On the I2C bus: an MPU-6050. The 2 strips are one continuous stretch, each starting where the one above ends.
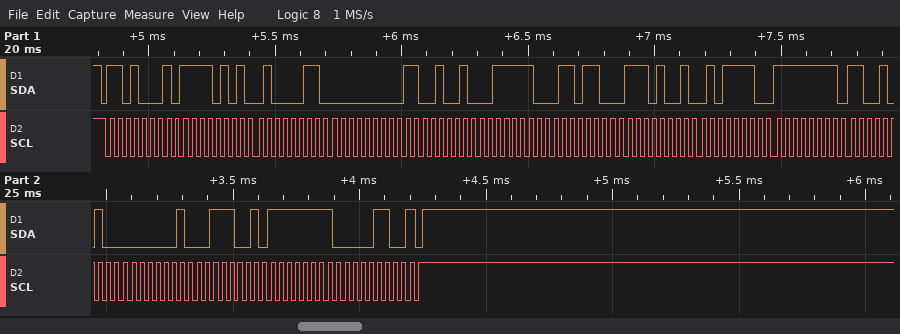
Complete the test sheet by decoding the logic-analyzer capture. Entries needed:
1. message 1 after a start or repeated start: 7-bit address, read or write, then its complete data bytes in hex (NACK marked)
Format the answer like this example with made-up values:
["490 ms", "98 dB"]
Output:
["0x68 read: F5 43 00 C9 3E 6C E9 5E FF CA 01 39 FF 0C NACK"]
